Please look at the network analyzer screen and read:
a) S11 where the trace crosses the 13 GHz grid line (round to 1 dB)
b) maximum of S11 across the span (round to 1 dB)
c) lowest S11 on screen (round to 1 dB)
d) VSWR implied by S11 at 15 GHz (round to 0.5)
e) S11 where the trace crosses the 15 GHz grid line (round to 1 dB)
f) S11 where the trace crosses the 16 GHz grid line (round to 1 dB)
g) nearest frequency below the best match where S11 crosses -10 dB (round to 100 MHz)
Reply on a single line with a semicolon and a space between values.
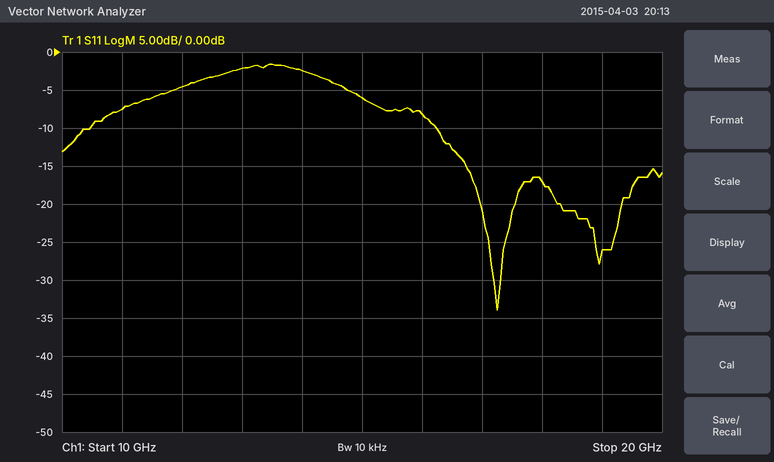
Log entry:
-2 dB; -2 dB; -34 dB; 3.0; -6 dB; -8 dB; 16.2 GHz
